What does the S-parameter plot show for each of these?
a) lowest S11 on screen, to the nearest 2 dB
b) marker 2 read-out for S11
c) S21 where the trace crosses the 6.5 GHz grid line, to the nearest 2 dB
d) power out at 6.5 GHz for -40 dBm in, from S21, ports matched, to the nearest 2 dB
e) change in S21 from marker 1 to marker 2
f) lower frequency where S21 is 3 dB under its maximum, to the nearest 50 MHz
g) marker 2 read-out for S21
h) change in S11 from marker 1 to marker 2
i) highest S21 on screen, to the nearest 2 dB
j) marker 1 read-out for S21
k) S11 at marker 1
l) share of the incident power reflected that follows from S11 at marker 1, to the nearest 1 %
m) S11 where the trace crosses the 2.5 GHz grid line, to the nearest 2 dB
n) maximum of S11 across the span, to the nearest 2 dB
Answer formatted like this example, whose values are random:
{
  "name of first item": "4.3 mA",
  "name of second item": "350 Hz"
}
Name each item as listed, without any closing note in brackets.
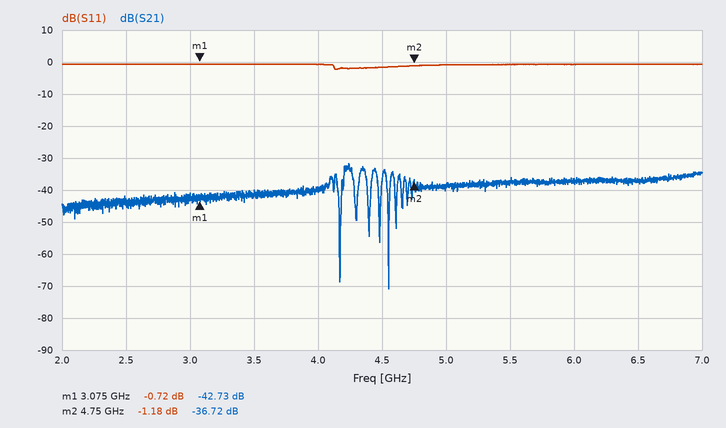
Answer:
{
  "lowest S11 on screen, to the nearest 2 dB": "-2 dB",
  "marker 2 read-out for S11": "-1.18 dB",
  "S21 where the trace crosses the 6.5 GHz grid line, to the nearest 2 dB": "-38 dB",
  "power out at 6.5 GHz for -40 dBm in, from S21, ports matched, to the nearest 2 dB": "-78 dBm",
  "change in S21 from marker 1 to marker 2": "6.01 dB",
  "lower frequency where S21 is 3 dB under its maximum, to the nearest 50 MHz": "4.20 GHz",
  "marker 2 read-out for S21": "-36.72 dB",
  "change in S11 from marker 1 to marker 2": "-0.46 dB",
  "highest S21 on screen, to the nearest 2 dB": "-32 dB",
  "marker 1 read-out for S21": "-42.73 dB",
  "S11 at marker 1": "-0.72 dB",
  "share of the incident power reflected that follows from S11 at marker 1, to the nearest 1 %": "85 %",
  "S11 where the trace crosses the 2.5 GHz grid line, to the nearest 2 dB": "0 dB",
  "maximum of S11 across the span, to the nearest 2 dB": "0 dB"
}
